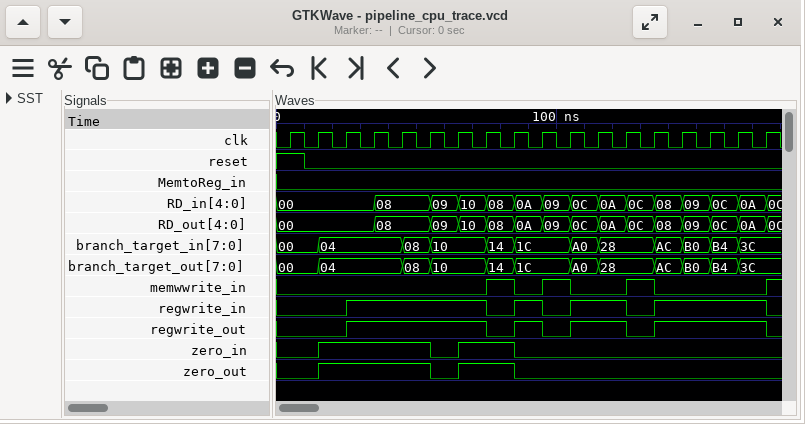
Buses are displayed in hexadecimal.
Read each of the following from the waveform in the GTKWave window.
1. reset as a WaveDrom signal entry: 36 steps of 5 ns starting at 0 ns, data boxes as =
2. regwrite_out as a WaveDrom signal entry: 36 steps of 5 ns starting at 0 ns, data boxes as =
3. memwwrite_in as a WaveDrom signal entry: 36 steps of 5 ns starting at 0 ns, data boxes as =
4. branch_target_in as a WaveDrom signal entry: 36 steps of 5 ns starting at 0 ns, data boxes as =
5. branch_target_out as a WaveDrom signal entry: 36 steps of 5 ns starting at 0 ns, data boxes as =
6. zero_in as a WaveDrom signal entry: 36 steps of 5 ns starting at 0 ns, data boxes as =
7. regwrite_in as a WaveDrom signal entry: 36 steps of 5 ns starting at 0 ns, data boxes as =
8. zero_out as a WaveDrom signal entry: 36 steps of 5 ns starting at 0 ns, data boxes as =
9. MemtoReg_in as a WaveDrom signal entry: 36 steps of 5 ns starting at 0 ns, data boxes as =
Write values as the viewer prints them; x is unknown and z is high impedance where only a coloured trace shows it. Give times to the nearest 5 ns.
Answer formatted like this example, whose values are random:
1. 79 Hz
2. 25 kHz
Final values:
1. {name: 'reset', wave: '1.0.................................'}
2. {name: 'regwrite_out', wave: '0....1.........0.1.0.1...0.1.......0'}
3. {name: 'memwwrite_in', wave: '0..............1.0.1.0...1.0.......1'}
4. {name: 'branch_target_in', wave: '=..=.....=.=...=.=...=.=...=.=.=.=..', data: '00 04 08 10 14 1C A0 28 AC B0 B4 3C'}
5. {name: 'branch_target_out', wave: '=..=.....=.=...=.=...=.=...=.=.=.=..', data: '00 04 08 10 14 1C A0 28 AC B0 B4 3C'}
6. {name: 'zero_in', wave: '0..1.......0.1...0..................'}
7. {name: 'regwrite_in', wave: '0....1.........0.1.0.1...0.1.......0'}
8. {name: 'zero_out', wave: '0..1.......0.1...0..................'}
9. {name: 'MemtoReg_in', wave: '0...................................'}
